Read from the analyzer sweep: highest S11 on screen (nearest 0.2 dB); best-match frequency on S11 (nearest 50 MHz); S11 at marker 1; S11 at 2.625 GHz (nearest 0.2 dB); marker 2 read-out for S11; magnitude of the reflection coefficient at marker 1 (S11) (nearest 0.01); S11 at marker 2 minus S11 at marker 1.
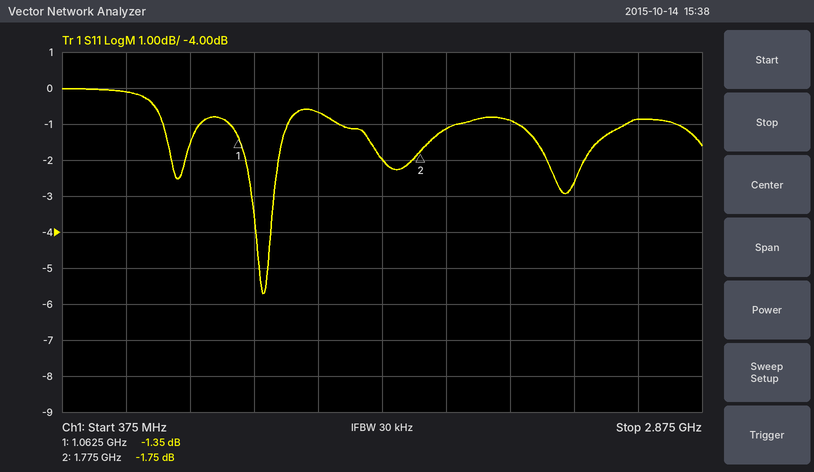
0.0 dB
1.15 GHz
-1.35 dB
-0.8 dB
-1.75 dB
0.86
-0.40 dB
